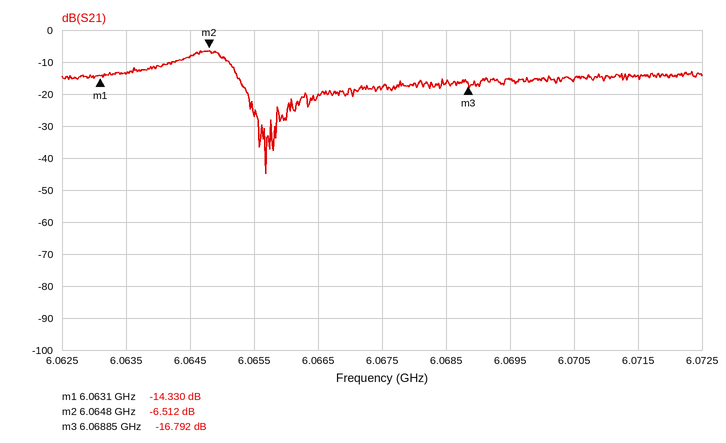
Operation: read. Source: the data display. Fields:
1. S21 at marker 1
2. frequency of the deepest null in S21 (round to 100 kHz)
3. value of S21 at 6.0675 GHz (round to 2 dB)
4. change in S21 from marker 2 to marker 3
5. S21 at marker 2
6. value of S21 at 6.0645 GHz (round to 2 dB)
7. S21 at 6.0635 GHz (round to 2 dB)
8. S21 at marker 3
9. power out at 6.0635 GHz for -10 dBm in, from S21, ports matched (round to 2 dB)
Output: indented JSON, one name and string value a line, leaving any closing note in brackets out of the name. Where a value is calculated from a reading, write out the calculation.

{
  "S21 at marker 1": "-14.330 dB",
  "frequency of the deepest null in S21": "6.0657 GHz",
  "value of S21 at 6.0675 GHz": "-18 dB",
  "change in S21 from marker 2 to marker 3": "-16.792 − (-6.512) = -10.280 dB",
  "S21 at marker 2": "-6.512 dB",
  "value of S21 at 6.0645 GHz": "-8 dB",
  "S21 at 6.0635 GHz": "-14 dB",
  "S21 at marker 3": "-16.792 dB",
  "power out at 6.0635 GHz for -10 dBm in, from S21, ports matched": "-10 dBm + (-14 dB) = -24 dBm"
}
